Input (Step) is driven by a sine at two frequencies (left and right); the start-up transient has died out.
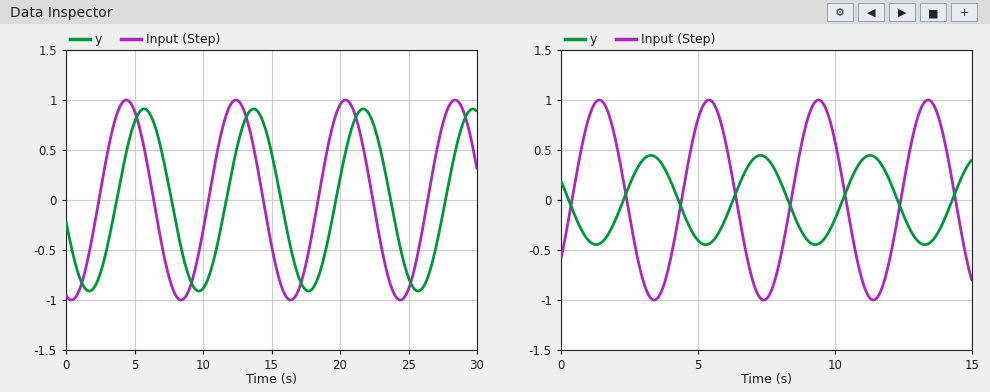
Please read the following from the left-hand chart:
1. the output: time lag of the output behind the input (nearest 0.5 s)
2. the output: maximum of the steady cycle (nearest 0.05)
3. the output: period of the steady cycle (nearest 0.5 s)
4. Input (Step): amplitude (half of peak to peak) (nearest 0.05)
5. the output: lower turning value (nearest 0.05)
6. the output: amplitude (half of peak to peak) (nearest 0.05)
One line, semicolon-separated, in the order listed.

1.5 s; 0.90; 8.0 s; 1.00; -0.90; 0.90
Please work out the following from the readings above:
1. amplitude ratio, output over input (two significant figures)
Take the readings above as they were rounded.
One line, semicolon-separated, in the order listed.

0.90
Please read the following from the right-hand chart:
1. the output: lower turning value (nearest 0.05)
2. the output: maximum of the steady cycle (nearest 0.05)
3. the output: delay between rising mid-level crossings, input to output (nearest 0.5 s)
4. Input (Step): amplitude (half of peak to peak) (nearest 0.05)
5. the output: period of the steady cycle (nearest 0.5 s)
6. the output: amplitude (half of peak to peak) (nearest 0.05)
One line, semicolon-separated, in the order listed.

-0.45; 0.45; 2.0 s; 1.00; 4.0 s; 0.45
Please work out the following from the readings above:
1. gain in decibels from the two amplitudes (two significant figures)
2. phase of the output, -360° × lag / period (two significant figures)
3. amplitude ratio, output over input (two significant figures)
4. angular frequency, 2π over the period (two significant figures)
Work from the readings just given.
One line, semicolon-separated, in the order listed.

-6.9 dB; -180°; 0.45; 1.6 rad/s
